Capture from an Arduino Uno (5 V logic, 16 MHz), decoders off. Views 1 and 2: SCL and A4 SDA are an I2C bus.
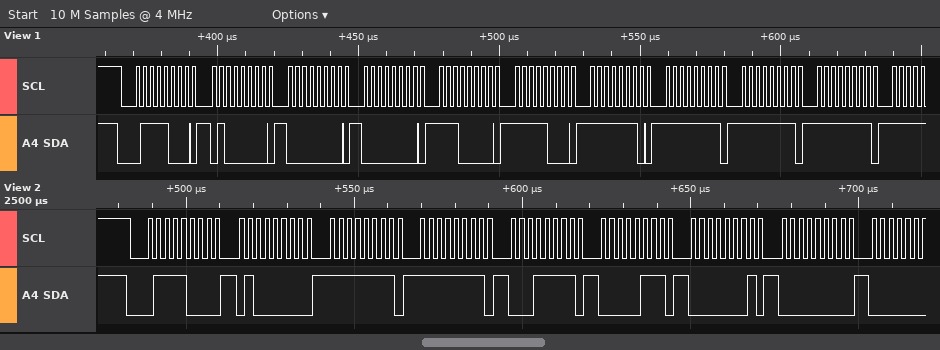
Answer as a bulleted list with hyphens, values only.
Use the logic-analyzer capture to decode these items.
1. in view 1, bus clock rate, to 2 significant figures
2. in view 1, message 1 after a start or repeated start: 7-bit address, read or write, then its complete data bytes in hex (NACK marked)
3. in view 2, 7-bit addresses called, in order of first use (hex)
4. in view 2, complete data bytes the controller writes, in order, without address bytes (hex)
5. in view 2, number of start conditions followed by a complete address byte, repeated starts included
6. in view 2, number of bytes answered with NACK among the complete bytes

- 400 kHz
- 0x3C write: 40 00 00 E0 F8 FE FF FF FF
- 0x3C
- 40 FF FF 1F 07 01 00
- 1
- 0
